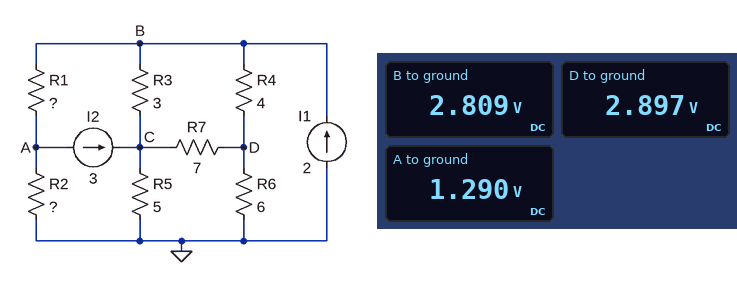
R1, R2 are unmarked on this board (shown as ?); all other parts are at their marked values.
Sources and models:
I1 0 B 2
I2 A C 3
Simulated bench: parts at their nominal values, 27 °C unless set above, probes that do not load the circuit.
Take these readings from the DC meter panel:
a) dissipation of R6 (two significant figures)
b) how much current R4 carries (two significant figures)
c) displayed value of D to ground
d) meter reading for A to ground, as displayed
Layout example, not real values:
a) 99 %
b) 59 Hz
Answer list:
a) 1.4 W
b) 22 mA
c) 2.897 V
d) 1.290 V
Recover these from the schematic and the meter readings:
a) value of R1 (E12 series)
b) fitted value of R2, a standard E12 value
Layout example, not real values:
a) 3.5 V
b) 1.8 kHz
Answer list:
a) 0.47 Ω
b) 5.6 Ω
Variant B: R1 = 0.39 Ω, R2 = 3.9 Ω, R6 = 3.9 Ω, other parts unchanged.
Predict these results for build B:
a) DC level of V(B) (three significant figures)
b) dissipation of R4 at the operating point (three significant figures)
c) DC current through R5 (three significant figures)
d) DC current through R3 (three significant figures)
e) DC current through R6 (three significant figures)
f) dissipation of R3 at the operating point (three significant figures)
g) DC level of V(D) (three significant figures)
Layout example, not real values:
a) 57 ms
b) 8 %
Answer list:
a) 2.22 V
b) 560 µW
c) 1.20 A
d) 1.26 A
e) 557 mA
f) 4.74 W
g) 2.17 V
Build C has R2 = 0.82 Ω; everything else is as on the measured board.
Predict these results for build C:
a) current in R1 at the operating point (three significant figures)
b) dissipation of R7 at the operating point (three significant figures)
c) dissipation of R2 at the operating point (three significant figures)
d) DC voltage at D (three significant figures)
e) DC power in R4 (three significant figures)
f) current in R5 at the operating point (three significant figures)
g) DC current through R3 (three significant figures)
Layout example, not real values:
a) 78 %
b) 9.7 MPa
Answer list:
a) 3.42 A
b) 1.77 W
c) 146 mW
d) 2.38 V
e) 45.3 mW
f) 1.18 A
g) 1.32 A
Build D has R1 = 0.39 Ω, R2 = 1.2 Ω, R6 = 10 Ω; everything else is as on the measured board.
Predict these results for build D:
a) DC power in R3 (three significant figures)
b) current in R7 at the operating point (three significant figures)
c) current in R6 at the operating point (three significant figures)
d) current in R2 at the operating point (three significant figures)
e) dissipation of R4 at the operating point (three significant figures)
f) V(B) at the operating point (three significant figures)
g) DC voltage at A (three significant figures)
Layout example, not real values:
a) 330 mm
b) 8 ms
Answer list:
a) 5.34 W
b) 464 mA
c) 276 mA
d) 523 mA
e) 142 mW
f) 2.00 V
g) 628 mV
